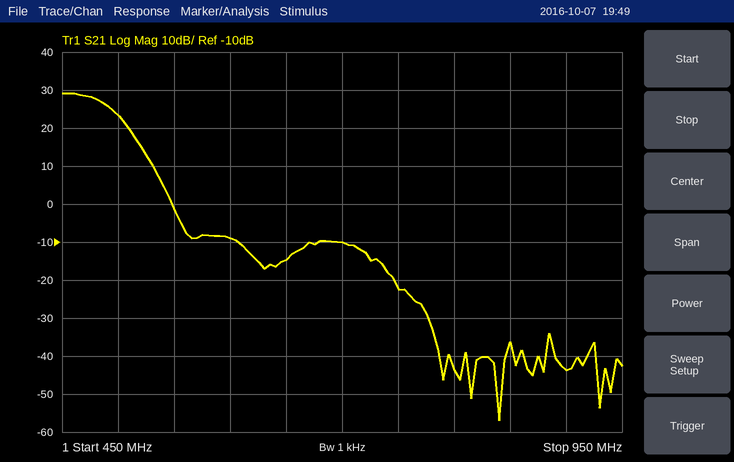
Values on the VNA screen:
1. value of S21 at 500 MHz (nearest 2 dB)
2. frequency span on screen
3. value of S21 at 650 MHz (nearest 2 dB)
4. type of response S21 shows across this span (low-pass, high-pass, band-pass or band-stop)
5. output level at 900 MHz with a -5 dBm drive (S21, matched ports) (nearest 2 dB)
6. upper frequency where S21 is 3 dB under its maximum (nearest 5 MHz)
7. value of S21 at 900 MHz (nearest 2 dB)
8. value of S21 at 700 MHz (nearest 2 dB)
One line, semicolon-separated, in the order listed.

24 dB; 500 MHz; -14 dB; low-pass; -48 dBm; 490 MHz; -44 dB; -10 dB
